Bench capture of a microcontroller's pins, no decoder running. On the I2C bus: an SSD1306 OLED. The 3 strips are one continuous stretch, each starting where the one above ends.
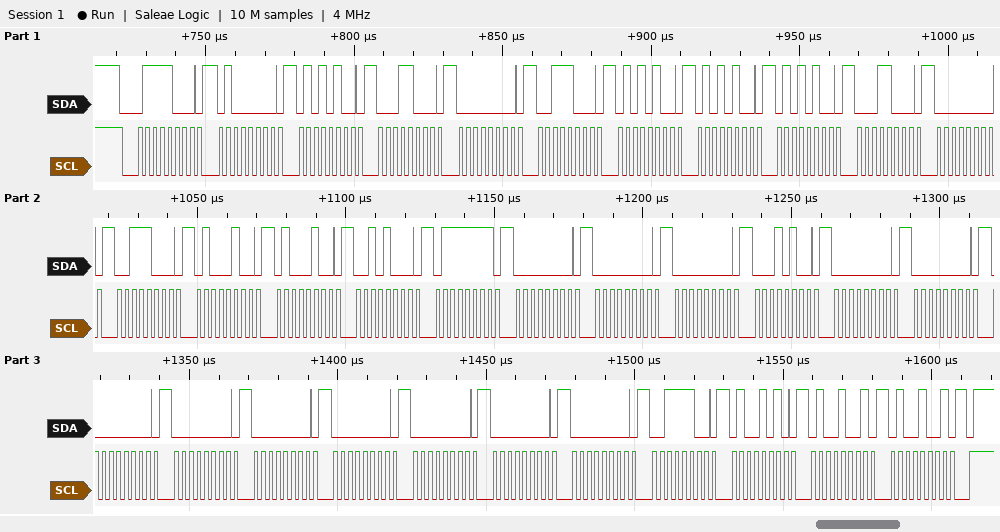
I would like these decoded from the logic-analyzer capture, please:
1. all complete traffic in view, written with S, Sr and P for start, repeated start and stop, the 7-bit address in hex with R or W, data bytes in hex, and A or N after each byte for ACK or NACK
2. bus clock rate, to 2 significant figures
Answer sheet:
S 3CW A 40 A 54 A 18 A 00 A 38 A 54 A 54 A 54 A 18 A 00 A 38 A 44 A 44 A 28 A 7F A 00 A 00 A 00 A 14 A 00 A 00 A 00 A 00 A 00 A 00 A 00 A 00 A 00 A 3C A 4A A 49 A 49 A P
400 kHz
